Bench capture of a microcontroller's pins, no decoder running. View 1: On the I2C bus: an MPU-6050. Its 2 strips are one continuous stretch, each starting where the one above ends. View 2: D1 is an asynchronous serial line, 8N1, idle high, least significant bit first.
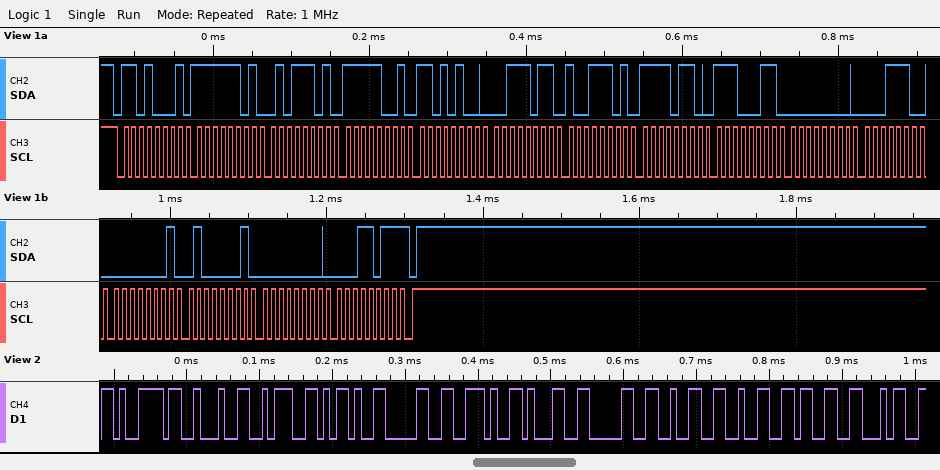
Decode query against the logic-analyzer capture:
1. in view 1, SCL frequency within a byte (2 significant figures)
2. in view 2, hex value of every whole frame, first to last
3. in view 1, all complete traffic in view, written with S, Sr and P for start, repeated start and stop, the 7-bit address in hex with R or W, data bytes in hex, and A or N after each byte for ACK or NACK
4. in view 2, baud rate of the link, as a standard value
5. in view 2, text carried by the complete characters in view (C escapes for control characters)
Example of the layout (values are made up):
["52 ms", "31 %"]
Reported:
["100 kHz", "0x79 0x22 0x3A 0x2D 0x30 0x2E 0x31 0x30 0x32 0x32 0x33 0x34", "S 68R A FD A 5D A F9 A D4 A 3B A 9D A F6 A E3 A 00 A 1C A 01 A 41 A 00 A 1B N P", "115200 baud", "\"y\\\":-0.102234\""]
